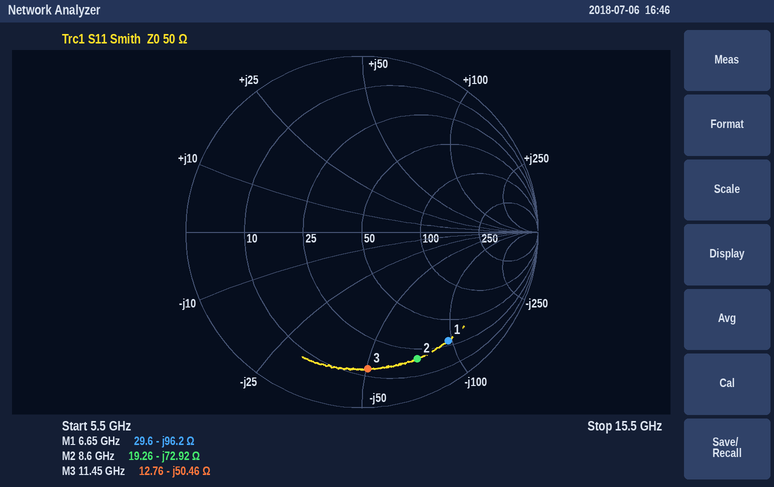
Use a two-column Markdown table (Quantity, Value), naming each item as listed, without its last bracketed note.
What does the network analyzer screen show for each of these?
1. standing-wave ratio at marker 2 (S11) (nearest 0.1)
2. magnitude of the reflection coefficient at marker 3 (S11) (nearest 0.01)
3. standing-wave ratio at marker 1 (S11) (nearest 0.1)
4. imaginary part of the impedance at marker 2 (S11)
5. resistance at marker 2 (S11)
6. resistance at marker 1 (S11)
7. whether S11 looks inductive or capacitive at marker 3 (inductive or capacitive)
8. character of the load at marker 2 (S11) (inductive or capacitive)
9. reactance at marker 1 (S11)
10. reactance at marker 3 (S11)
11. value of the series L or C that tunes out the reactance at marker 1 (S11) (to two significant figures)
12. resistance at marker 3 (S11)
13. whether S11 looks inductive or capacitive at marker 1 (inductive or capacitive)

| Quantity | Value |
|---|---|
| standing-wave ratio at marker 2 (S11) | 8.4 |
| magnitude of the reflection coefficient at marker 3 (S11) | 0.78 |
| standing-wave ratio at marker 1 (S11) | 8.4 |
| imaginary part of the impedance at marker 2 | -72.92 Ω |
| resistance at marker 2 | 19.26 Ω |
| resistance at marker 1 | 29.6 Ω |
| whether S11 looks inductive or capacitive at marker 3 | capacitive |
| character of the load at marker 2 (S11) | capacitive |
| reactance at marker 1 | -96.2 Ω |
| reactance at marker 3 | -50.46 Ω |
| value of the series L or C that tunes out the reactance at marker 1 (S11) | 2.3 nH |
| resistance at marker 3 | 12.76 Ω |
| whether S11 looks inductive or capacitive at marker 1 | capacitive |
